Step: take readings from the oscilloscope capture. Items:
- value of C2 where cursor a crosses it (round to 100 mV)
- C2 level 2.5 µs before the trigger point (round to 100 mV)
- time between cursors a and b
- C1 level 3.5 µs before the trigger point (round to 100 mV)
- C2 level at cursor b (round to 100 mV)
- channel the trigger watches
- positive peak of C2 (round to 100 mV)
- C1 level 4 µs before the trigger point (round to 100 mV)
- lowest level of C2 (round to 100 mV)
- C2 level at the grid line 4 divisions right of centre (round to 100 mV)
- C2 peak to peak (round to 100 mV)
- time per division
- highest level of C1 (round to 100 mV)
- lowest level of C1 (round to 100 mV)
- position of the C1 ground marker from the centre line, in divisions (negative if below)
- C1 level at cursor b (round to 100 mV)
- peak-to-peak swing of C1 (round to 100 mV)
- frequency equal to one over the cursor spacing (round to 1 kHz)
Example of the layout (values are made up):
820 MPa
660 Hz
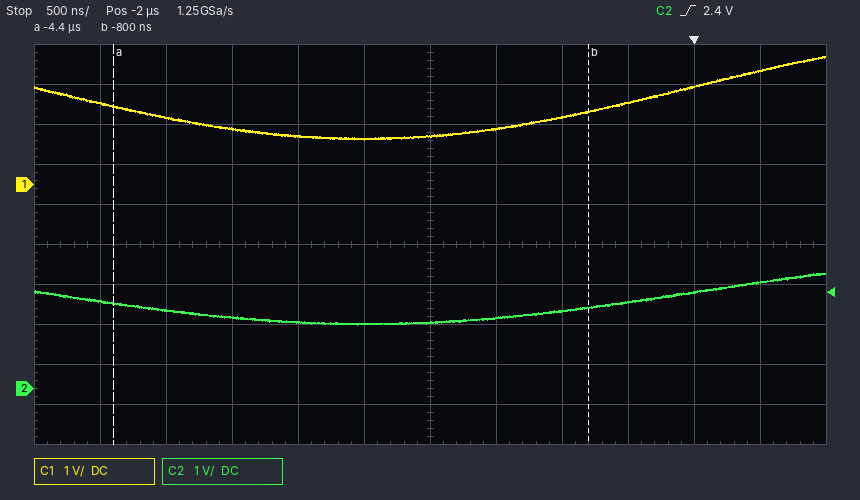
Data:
2.1 V
1.6 V
3.60 µs
1.4 V
2.0 V
C2
2.9 V
1.7 V
1.6 V
2.4 V
1.3 V
500 ns
3.2 V
1.1 V
+1.5 div
1.8 V
2.1 V
278 kHz
